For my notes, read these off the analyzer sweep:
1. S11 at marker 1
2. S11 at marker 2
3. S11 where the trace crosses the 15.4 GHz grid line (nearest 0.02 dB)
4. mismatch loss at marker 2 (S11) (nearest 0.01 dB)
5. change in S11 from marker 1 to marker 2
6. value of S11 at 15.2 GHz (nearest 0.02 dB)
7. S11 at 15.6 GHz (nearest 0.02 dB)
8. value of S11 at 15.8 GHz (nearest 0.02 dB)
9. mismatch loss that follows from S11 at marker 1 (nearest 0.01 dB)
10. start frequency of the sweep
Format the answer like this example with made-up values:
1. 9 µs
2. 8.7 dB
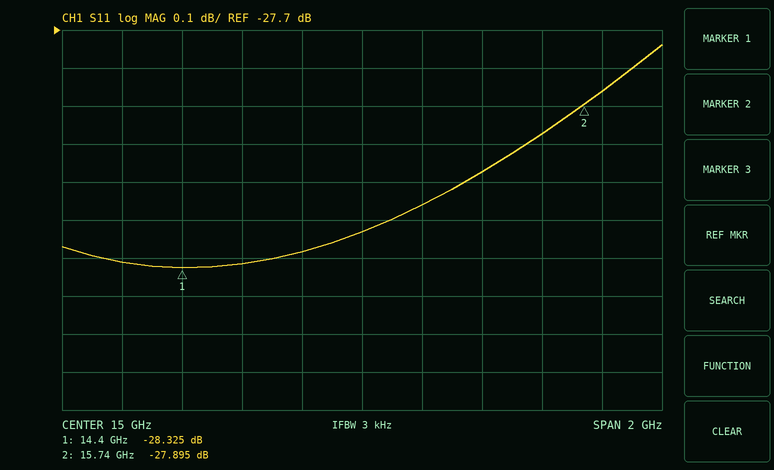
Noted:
1. -28.325 dB
2. -27.895 dB
3. -28.08 dB
4. 0.01 dB
5. 0.430 dB
6. -28.16 dB
7. -27.98 dB
8. -27.86 dB
9. 0.01 dB
10. 14 GHz
